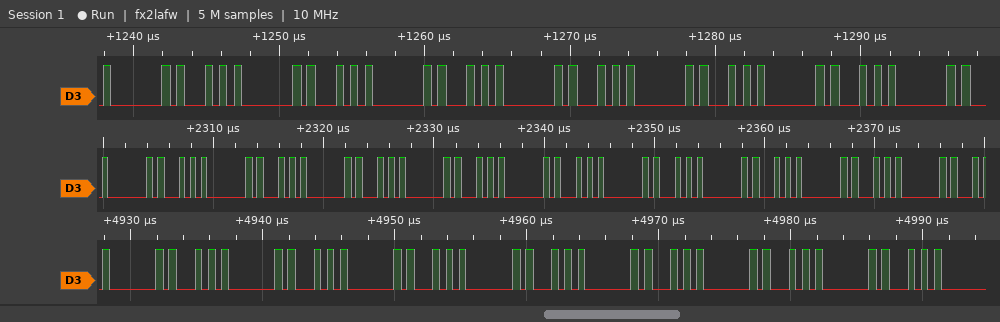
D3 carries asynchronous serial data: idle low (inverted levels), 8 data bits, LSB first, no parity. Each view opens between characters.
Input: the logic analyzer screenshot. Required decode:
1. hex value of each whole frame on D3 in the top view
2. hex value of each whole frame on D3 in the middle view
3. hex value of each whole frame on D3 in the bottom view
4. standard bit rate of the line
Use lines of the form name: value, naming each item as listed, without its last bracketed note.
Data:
hex value of each whole frame on D3 in the top view: 7F, 57, 5D, 7F, 57, 5D, 7F, 57, 5D, 7F
hex value of each whole frame on D3 in the middle view: 7F, 57, 5D, 7F, 57, 5D, 7F, 57, 5D, 7F, 57, 5D, 7F
hex value of each whole frame on D3 in the bottom view: 7F, 57, 5D, 7F, 57, 5D, 7F, 57, 5D, 7F, 57
standard bit rate of the line: 2000000 baud
